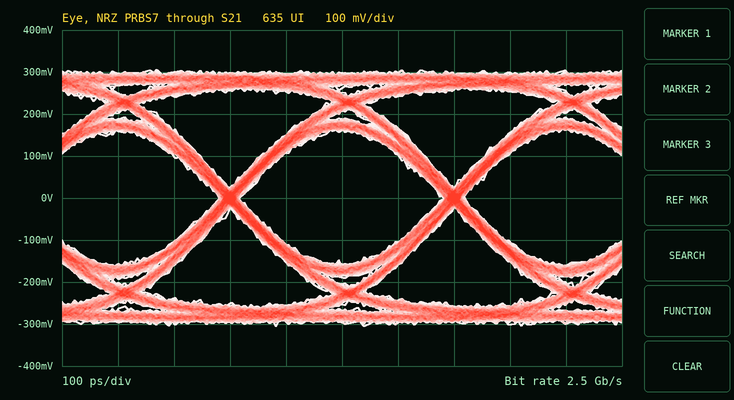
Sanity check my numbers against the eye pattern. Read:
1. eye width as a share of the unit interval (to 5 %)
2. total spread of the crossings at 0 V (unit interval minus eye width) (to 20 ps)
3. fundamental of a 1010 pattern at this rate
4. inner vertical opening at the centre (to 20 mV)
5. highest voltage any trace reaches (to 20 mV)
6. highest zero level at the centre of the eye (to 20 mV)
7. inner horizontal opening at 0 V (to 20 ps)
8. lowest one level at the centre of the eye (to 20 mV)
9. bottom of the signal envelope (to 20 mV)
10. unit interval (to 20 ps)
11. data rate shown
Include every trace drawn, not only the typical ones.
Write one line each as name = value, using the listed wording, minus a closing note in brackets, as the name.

eye width as a share of the unit interval = 90 %
total spread of the crossings at 0 V (unit interval minus eye width) = 40 ps
fundamental of a 1010 pattern at this rate = 1.25 GHz
inner vertical opening at the centre = 320 mV
highest voltage any trace reaches = 300 mV
highest zero level at the centre of the eye = -160 mV
inner horizontal opening at 0 V = 360 ps
lowest one level at the centre of the eye = 160 mV
bottom of the signal envelope = -300 mV
unit interval = 400 ps
data rate shown = 2.5 Gb/s
